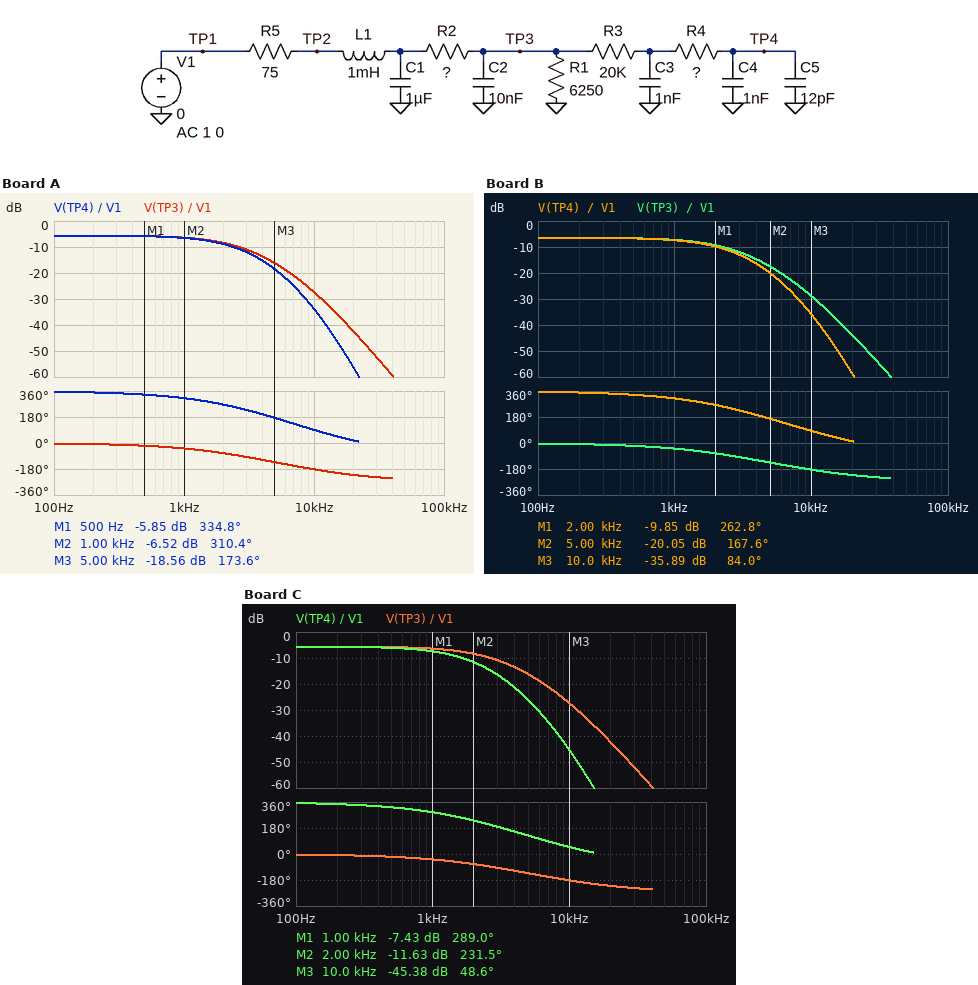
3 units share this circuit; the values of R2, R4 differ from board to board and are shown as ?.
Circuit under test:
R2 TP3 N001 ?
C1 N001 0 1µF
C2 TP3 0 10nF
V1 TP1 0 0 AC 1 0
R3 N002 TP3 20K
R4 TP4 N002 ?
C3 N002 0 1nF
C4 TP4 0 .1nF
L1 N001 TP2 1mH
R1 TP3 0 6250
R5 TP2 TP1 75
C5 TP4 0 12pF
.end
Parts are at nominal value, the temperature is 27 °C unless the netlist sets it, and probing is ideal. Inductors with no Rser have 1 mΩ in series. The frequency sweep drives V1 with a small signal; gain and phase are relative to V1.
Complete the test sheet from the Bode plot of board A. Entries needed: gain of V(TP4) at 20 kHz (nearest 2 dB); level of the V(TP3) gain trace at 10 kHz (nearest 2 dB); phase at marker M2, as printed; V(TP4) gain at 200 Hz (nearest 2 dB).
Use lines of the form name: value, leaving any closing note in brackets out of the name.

gain of V(TP4) at 20 kHz: -56 dB
level of the V(TP3) gain trace at 10 kHz: -28 dB
phase at marker M2, as printed: 310.4 deg
V(TP4) gain at 200 Hz: -6 dB
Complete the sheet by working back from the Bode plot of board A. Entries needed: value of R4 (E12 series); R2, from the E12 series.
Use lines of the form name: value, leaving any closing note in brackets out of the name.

value of R4: 100 kΩ
R2, from the E12 series: 5.6 kΩ
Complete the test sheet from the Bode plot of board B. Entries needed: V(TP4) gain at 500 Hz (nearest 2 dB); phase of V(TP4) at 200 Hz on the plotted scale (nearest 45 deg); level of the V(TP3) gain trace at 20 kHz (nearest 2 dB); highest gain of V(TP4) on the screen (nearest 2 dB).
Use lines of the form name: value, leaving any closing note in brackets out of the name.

V(TP4) gain at 500 Hz: -6 dB
phase of V(TP4) at 200 Hz on the plotted scale: 360 deg
level of the V(TP3) gain trace at 20 kHz: -44 dB
highest gain of V(TP4) on the screen: -6 dB
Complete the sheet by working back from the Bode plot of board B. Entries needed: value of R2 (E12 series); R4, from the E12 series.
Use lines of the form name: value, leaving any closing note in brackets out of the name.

value of R2: 6.8 kΩ
R4, from the E12 series: 120 kΩ
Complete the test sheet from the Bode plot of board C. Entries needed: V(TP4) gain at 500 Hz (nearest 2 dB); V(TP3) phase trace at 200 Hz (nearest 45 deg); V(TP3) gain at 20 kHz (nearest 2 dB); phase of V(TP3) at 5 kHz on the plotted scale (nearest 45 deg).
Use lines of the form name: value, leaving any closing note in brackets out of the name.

V(TP4) gain at 500 Hz: -6 dB
V(TP3) phase trace at 200 Hz: 0 deg
V(TP3) gain at 20 kHz: -42 dB
phase of V(TP3) at 5 kHz on the plotted scale: -135 deg
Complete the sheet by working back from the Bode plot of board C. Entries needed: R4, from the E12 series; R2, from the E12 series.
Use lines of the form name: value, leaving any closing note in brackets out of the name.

R4, from the E12 series: 680 kΩ
R2, from the E12 series: 5.6 kΩ
